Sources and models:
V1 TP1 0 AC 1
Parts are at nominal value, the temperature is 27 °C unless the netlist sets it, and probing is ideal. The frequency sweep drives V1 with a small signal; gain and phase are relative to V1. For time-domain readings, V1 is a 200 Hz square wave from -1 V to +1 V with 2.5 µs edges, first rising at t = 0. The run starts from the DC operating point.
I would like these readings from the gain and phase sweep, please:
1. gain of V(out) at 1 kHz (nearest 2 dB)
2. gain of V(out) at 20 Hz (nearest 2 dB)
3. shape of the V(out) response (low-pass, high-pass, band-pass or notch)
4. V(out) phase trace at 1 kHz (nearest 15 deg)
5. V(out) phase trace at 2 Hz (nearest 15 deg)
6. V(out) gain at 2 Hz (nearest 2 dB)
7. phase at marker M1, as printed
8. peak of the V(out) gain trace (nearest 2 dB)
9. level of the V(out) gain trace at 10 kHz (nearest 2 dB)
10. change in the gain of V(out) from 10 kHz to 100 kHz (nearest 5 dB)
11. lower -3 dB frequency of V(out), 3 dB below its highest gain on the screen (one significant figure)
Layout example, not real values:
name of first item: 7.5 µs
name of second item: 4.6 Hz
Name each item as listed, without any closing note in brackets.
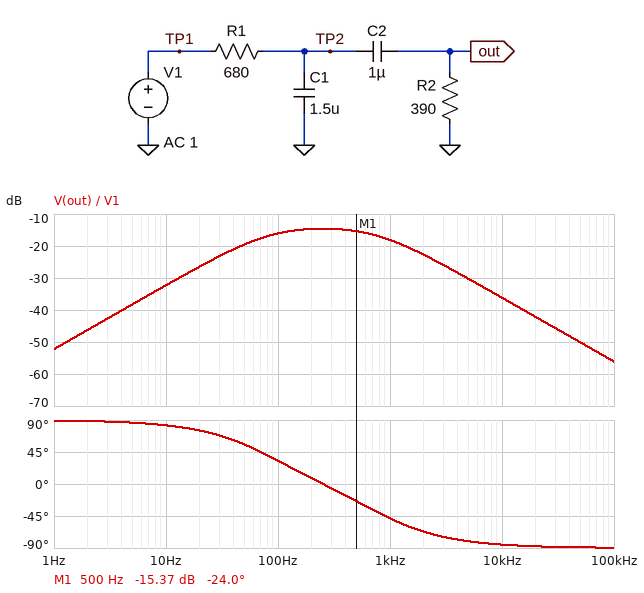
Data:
gain of V(out) at 1 kHz: -18 dB
gain of V(out) at 20 Hz: -26 dB
shape of the V(out) response: band-pass
V(out) phase trace at 1 kHz: -45 deg
V(out) phase trace at 2 Hz: 90 deg
V(out) gain at 2 Hz: -46 dB
phase at marker M1, as printed: -24.0 deg
peak of the V(out) gain trace: -14 dB
level of the V(out) gain trace at 10 kHz: -36 dB
change in the gain of V(out) from 10 kHz to 100 kHz: -20 dB
lower -3 dB frequency of V(out), 3 dB below its highest gain on the screen: 70 Hz
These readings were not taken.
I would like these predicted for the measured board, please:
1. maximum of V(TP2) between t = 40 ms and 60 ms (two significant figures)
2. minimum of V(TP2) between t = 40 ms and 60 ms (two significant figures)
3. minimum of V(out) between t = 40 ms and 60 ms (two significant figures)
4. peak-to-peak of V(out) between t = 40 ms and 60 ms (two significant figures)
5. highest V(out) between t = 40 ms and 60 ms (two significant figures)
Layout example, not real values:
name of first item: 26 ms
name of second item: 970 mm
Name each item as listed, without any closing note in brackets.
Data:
maximum of V(TP2) between t = 40 ms and 60 ms: 630 mV
minimum of V(TP2) between t = 40 ms and 60 ms: -630 mV
minimum of V(out) between t = 40 ms and 60 ms: -240 mV
peak-to-peak of V(out) between t = 40 ms and 60 ms: 480 mV
highest V(out) between t = 40 ms and 60 ms: 240 mV
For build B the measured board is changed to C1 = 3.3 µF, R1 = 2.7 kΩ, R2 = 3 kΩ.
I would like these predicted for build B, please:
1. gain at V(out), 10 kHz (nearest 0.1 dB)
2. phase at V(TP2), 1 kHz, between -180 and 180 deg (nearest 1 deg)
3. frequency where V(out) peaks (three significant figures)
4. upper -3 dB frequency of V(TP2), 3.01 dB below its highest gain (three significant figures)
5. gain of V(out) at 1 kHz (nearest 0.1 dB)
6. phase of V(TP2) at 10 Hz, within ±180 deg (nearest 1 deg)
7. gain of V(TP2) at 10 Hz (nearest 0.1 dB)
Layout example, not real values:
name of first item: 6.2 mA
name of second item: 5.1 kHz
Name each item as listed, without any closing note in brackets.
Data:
gain at V(out), 10 kHz: -55.0 dB
phase at V(TP2), 1 kHz, between -180 and 180 deg: -88 deg
frequency where V(out) peaks: 30.8 Hz
upper -3 dB frequency of V(TP2), 3.01 dB below its highest gain: 13.1 Hz
gain of V(out) at 1 kHz: -35.0 dB
phase of V(TP2) at 10 Hz, within ±180 deg: -35 deg
gain of V(TP2) at 10 Hz: -2.0 dB
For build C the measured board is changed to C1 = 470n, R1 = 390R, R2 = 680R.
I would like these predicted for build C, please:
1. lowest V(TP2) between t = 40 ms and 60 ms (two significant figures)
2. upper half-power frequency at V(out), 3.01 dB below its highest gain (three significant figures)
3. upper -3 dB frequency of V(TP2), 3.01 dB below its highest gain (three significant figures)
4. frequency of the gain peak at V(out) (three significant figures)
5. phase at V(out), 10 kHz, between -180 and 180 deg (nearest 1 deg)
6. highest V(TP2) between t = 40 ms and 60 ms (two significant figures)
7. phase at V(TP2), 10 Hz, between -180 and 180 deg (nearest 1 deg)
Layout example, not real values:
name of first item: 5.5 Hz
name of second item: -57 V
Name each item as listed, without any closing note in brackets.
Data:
lowest V(TP2) between t = 40 ms and 60 ms: -910 mV
upper half-power frequency at V(out), 3.01 dB below its highest gain: 1.72 kHz
upper -3 dB frequency of V(TP2), 3.01 dB below its highest gain: 242 Hz
frequency of the gain peak at V(out): 451 Hz
phase at V(out), 10 kHz, between -180 and 180 deg: -81 deg
highest V(TP2) between t = 40 ms and 60 ms: 910 mV
phase at V(TP2), 10 Hz, between -180 and 180 deg: -2 deg
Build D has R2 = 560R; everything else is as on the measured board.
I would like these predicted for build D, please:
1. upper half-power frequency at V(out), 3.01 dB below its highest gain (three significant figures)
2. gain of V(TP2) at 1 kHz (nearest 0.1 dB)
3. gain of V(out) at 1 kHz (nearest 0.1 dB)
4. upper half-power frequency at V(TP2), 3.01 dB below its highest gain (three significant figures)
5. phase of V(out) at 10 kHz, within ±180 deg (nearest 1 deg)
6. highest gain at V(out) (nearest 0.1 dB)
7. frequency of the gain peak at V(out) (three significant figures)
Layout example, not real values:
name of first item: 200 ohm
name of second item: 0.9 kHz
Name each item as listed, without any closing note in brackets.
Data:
upper half-power frequency at V(out), 3.01 dB below its highest gain: 694 Hz
gain of V(TP2) at 1 kHz: -17.0 dB
gain of V(out) at 1 kHz: -17.3 dB
upper half-power frequency at V(TP2), 3.01 dB below its highest gain: 85.9 Hz
phase of V(out) at 10 kHz, within ±180 deg: -86 deg
highest gain at V(out): -12.1 dB
frequency of the gain peak at V(out): 211 Hz
